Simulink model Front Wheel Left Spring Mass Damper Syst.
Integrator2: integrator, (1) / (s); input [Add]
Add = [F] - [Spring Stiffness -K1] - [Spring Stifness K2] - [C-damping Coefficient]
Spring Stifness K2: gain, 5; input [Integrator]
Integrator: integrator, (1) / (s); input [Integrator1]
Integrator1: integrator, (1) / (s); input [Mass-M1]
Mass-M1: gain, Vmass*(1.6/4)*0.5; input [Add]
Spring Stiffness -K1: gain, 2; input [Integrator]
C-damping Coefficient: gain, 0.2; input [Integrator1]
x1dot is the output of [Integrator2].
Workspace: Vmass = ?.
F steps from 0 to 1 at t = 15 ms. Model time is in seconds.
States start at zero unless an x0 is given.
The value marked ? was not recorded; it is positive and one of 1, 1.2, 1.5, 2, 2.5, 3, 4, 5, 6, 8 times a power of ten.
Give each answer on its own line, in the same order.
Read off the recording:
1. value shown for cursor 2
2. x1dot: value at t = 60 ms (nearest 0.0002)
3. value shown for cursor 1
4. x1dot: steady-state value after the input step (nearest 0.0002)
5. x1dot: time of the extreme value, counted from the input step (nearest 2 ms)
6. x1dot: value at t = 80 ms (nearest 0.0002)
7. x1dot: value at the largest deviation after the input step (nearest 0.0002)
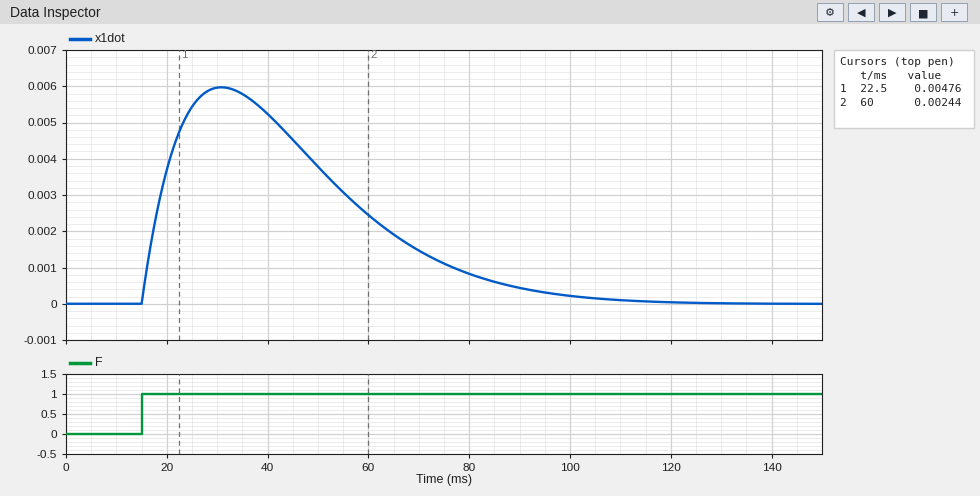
0.00244
0.0024
0.00476
0.0000
16 ms
0.0008
0.0060
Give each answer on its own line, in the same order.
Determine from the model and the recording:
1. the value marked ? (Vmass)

3000
